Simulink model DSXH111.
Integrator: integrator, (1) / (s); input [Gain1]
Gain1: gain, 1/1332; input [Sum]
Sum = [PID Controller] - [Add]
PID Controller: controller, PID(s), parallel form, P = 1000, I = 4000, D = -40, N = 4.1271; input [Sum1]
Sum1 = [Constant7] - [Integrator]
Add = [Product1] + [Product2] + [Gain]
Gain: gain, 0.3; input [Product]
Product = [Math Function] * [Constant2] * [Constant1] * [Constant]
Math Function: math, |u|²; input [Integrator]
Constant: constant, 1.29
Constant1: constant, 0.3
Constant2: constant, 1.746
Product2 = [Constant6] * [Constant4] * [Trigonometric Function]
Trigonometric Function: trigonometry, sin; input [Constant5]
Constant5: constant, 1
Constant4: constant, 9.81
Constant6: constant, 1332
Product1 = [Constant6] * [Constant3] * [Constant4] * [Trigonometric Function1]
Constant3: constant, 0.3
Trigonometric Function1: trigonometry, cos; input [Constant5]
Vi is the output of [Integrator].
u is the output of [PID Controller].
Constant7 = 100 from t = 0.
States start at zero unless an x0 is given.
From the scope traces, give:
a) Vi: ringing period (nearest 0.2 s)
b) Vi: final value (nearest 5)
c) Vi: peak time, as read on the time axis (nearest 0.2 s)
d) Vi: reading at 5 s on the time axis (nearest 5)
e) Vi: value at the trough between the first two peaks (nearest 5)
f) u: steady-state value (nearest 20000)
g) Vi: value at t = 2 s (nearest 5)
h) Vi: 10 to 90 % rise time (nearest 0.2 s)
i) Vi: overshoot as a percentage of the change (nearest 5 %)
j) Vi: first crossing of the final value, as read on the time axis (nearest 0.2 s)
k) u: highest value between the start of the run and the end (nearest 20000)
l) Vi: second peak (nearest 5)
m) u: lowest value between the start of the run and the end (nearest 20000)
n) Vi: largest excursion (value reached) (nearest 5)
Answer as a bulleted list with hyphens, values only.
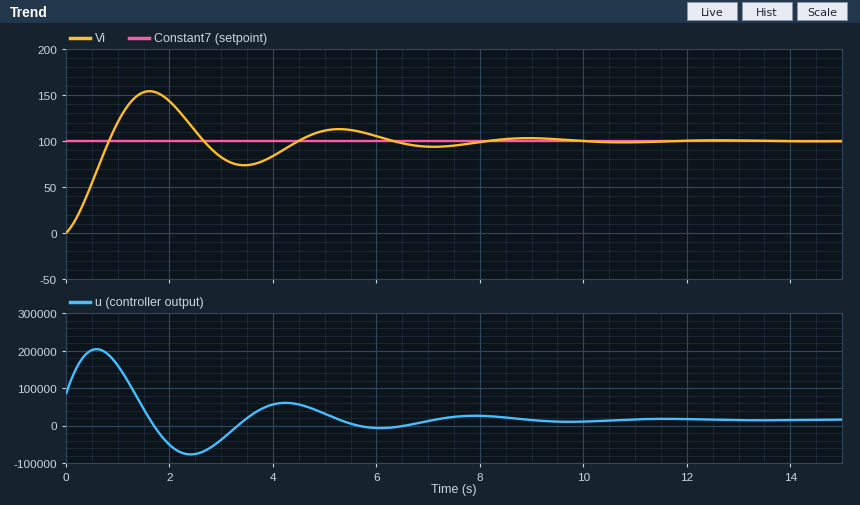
- 3.6 s
- 100
- 1.6 s
- 110
- 75
- 20000
- 145
- 0.6 s
- 55 %
- 0.8 s
- 200000
- 115
- -80000
- 155
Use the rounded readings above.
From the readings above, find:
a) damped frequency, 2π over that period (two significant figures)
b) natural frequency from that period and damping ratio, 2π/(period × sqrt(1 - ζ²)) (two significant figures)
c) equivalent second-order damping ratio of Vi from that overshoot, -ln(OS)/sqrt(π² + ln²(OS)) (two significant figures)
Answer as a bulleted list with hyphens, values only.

- 1.7 rad/s
- 1.8 rad/s
- 0.19
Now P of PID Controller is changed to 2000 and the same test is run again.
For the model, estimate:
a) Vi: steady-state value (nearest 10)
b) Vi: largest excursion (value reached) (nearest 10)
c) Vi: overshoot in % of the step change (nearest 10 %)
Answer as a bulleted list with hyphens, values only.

- 100
- 130
- 30 %
